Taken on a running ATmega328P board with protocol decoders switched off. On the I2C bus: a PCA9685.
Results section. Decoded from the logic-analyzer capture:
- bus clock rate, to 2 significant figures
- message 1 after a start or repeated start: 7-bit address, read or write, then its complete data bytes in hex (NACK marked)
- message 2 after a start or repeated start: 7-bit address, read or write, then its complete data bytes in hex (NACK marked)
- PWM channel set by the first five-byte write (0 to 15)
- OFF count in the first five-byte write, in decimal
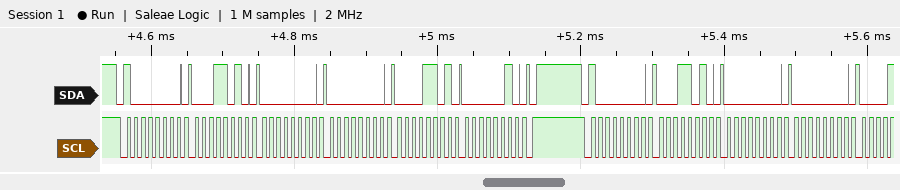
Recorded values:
100 kHz
0x40 write: 1A 00 00 0D 02
0x40 write: 1A 00 00
5
525
